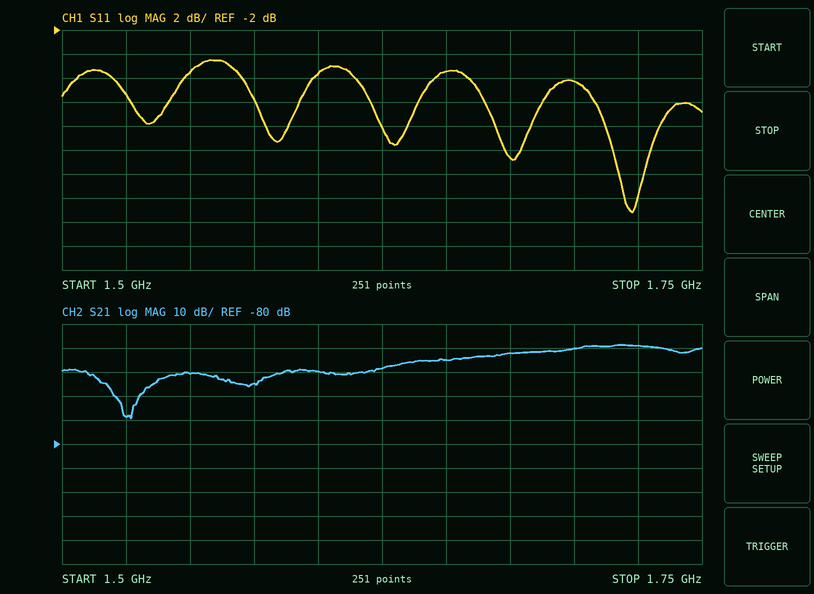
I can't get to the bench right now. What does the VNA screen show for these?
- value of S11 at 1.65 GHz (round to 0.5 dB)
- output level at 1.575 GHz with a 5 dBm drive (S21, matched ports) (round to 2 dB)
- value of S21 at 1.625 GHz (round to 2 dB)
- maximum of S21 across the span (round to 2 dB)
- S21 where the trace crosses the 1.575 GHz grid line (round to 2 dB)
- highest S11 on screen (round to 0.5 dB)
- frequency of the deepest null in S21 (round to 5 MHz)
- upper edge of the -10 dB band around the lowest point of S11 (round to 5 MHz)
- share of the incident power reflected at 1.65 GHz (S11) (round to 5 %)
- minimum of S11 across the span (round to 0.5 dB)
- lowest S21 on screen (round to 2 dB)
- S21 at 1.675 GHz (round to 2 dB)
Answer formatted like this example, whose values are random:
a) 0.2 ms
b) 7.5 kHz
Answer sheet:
a) -5.5 dB
b) -50 dBm
c) -48 dB
d) -38 dB
e) -54 dB
f) -4.5 dB
g) 1.525 GHz
h) 1.735 GHz
i) 30 %
j) -17.0 dB
k) -70 dB
l) -42 dB
